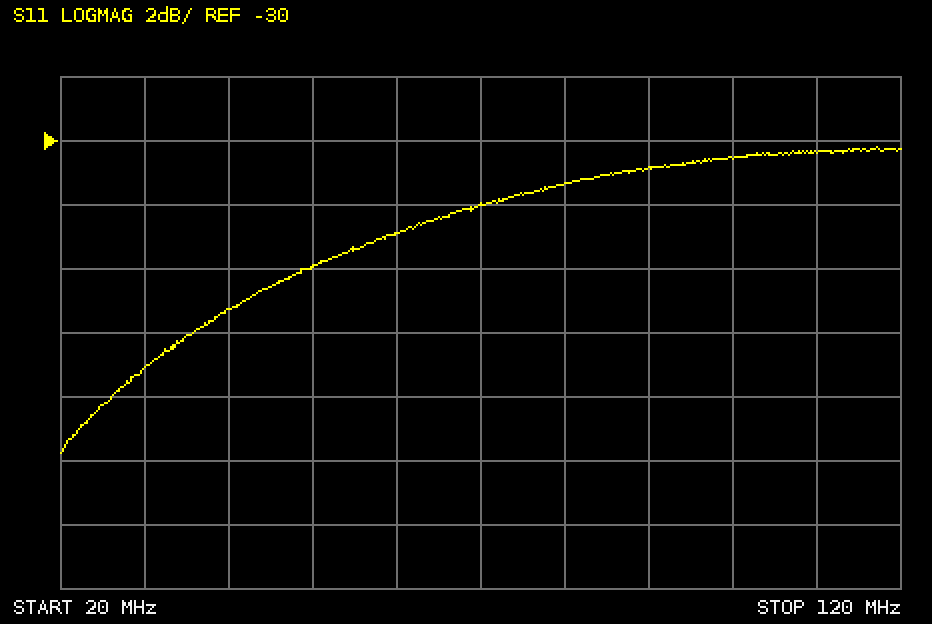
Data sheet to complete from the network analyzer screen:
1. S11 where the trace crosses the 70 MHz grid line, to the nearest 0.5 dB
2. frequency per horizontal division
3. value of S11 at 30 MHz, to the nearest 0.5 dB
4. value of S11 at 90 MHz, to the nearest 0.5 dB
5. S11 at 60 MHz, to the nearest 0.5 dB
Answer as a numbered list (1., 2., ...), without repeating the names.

1. -32.0 dB
2. 10 MHz
3. -37.0 dB
4. -31.0 dB
5. -33.0 dB
